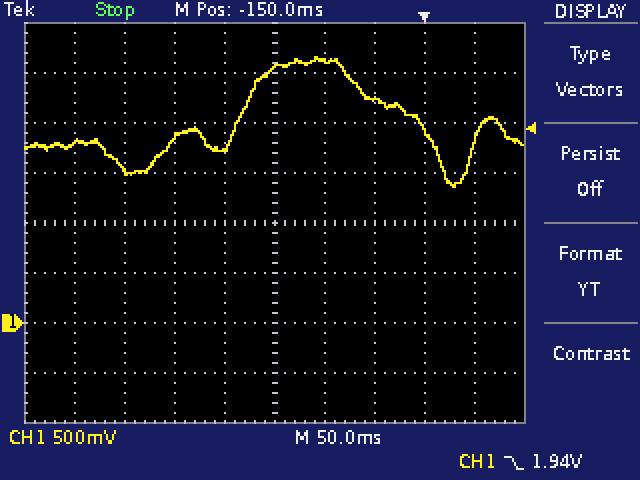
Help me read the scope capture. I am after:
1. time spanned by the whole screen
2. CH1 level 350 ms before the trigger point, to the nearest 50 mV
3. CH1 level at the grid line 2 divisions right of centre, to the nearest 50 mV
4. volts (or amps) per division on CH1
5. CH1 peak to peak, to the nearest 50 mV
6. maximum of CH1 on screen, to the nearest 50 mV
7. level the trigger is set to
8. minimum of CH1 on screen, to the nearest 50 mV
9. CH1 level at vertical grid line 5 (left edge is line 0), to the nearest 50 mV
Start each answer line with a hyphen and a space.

- 500 ms
- 1.80 V
- 2.25 V
- 500 mV
- 1.30 V
- 2.65 V
- 1.94 V
- 1.35 V
- 2.55 V
